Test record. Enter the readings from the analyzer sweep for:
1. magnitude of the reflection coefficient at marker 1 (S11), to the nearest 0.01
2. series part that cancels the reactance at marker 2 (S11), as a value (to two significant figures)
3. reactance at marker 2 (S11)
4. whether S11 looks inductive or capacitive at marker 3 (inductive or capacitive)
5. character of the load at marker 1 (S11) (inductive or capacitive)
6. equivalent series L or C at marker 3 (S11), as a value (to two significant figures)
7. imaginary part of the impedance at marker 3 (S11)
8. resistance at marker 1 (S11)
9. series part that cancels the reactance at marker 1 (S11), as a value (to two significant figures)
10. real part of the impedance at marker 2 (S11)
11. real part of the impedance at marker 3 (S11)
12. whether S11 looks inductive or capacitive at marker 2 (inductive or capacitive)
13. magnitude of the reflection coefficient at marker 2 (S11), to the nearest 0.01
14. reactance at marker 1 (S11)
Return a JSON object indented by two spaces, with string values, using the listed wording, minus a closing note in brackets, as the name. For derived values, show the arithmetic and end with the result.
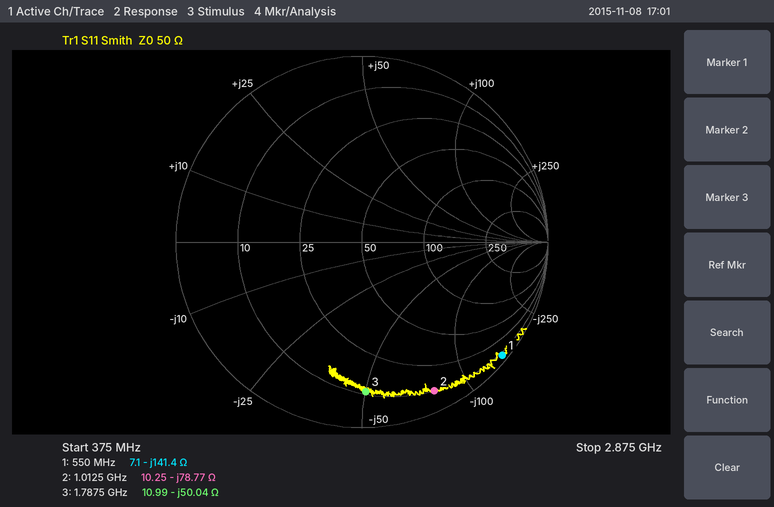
{
  "magnitude of the reflection coefficient at marker 1 (S11), to the nearest 0.01": "0.97",
  "series part that cancels the reactance at marker 2 (S11), as a value": "L = 78.77 Ω/(2π × 1.0125 GHz) ≈ 12 nH",
  "reactance at marker 2": "-78.77 Ω",
  "whether S11 looks inductive or capacitive at marker 3": "capacitive",
  "character of the load at marker 1 (S11)": "capacitive",
  "equivalent series L or C at marker 3 (S11), as a value": "C = 1/(2π × 1.7875 GHz × 50.04 Ω) ≈ 1.8 pF",
  "imaginary part of the impedance at marker 3": "-50.04 Ω",
  "resistance at marker 1": "7.1 Ω",
  "series part that cancels the reactance at marker 1 (S11), as a value": "L = 141.4 Ω/(2π × 550 MHz) ≈ 41 nH",
  "real part of the impedance at marker 2": "10.25 Ω",
  "real part of the impedance at marker 3": "10.99 Ω",
  "whether S11 looks inductive or capacitive at marker 2": "capacitive",
  "magnitude of the reflection coefficient at marker 2 (S11), to the nearest 0.01": "0.89",
  "reactance at marker 1": "-141.4 Ω"
}
